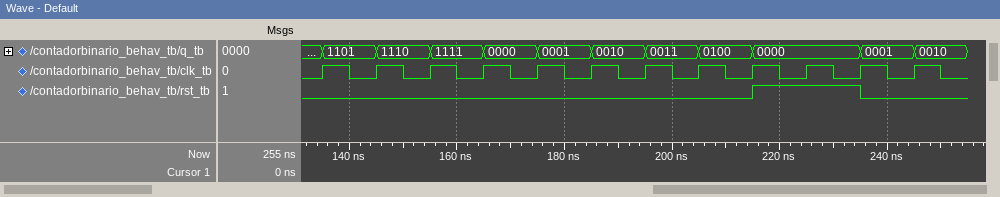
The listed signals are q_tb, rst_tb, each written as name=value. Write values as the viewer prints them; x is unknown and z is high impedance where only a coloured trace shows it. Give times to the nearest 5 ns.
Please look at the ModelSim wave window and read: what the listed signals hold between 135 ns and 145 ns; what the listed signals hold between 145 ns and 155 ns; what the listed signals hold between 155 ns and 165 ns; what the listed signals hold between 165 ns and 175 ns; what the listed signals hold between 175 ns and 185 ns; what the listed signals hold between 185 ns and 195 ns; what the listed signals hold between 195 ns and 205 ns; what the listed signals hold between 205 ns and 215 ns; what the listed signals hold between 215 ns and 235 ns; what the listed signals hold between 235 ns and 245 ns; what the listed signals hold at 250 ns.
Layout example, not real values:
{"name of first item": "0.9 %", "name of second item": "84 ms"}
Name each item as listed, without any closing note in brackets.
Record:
{"what the listed signals hold between 135 ns and 145 ns": "q_tb=1101, rst_tb=0", "what the listed signals hold between 145 ns and 155 ns": "q_tb=1110, rst_tb=0", "what the listed signals hold between 155 ns and 165 ns": "q_tb=1111, rst_tb=0", "what the listed signals hold between 165 ns and 175 ns": "q_tb=0000, rst_tb=0", "what the listed signals hold between 175 ns and 185 ns": "q_tb=0001, rst_tb=0", "what the listed signals hold between 185 ns and 195 ns": "q_tb=0010, rst_tb=0", "what the listed signals hold between 195 ns and 205 ns": "q_tb=0011, rst_tb=0", "what the listed signals hold between 205 ns and 215 ns": "q_tb=0100, rst_tb=0", "what the listed signals hold between 215 ns and 235 ns": "q_tb=0000, rst_tb=1", "what the listed signals hold between 235 ns and 245 ns": "q_tb=0001, rst_tb=0", "what the listed signals hold at 250 ns": "q_tb=0010, rst_tb=0"}
